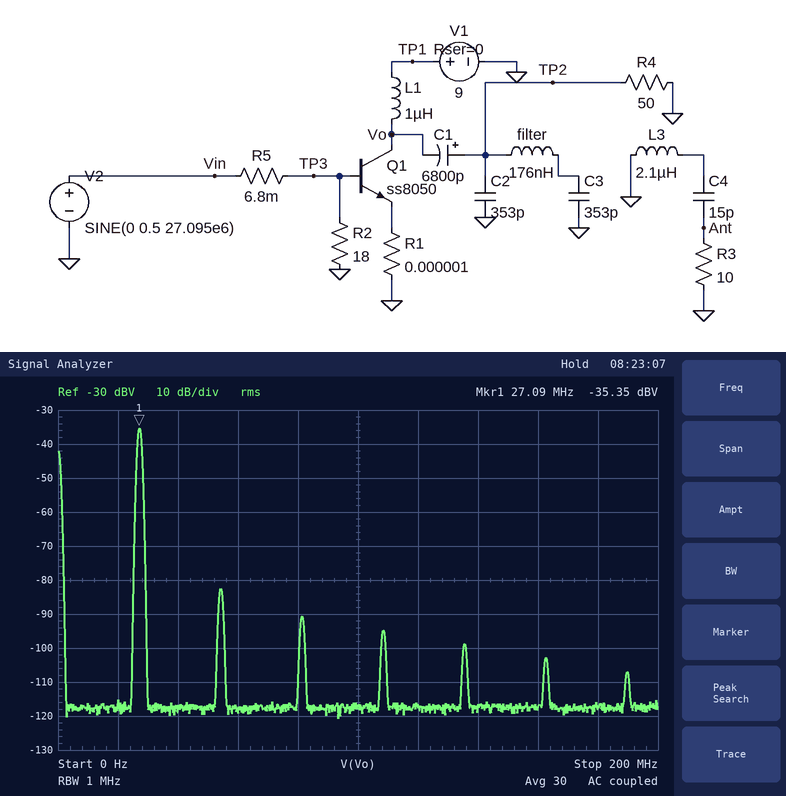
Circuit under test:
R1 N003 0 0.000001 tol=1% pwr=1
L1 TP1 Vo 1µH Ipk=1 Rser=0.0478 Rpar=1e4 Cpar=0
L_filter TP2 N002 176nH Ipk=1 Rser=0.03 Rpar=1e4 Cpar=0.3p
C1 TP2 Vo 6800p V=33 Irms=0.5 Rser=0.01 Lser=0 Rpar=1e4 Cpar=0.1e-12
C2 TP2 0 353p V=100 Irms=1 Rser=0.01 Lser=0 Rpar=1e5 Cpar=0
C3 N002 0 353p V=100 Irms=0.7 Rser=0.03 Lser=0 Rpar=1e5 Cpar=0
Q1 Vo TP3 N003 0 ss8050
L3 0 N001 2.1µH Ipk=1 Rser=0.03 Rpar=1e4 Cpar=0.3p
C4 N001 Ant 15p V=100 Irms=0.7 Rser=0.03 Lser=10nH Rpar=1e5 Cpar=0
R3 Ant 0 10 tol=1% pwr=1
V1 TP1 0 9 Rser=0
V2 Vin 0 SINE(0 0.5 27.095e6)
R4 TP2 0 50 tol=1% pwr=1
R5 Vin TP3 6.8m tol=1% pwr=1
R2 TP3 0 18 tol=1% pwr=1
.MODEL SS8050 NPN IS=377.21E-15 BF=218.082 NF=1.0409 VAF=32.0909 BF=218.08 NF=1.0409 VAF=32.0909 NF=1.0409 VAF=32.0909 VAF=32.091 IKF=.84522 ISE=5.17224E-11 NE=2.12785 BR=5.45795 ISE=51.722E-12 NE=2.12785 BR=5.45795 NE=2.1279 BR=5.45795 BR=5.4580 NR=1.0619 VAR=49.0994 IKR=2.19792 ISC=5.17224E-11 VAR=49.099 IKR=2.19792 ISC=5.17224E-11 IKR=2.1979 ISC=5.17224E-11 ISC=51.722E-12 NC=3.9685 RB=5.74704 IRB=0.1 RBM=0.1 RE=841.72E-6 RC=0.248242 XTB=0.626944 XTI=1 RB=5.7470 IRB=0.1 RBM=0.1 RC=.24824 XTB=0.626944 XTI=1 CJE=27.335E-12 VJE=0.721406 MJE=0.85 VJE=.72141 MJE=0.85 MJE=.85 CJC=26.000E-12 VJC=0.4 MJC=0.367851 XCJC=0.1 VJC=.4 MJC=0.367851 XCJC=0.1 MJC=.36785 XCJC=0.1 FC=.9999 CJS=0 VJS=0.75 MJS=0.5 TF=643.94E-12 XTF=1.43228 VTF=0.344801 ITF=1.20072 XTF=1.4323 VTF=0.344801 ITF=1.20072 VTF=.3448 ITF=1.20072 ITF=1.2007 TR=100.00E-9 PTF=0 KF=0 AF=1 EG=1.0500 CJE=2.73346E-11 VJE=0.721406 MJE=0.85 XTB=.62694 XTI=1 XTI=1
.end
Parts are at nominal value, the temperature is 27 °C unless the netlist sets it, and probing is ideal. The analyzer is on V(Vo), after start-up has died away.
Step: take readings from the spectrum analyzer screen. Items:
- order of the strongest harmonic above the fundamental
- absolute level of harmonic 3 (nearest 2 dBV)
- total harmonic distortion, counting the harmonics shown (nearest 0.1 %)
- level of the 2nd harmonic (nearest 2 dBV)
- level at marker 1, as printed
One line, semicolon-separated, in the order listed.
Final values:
2; -90 dBV; 0.5 %; -82 dBV; -35.35 dBV
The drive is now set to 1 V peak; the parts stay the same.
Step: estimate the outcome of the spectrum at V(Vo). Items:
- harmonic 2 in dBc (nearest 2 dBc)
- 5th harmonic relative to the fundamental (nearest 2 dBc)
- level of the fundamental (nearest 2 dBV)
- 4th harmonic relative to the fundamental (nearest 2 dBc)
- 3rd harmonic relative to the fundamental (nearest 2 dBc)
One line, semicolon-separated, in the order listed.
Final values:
-16 dBc; -34 dBc; 6 dBV; -34 dBc; -34 dBc
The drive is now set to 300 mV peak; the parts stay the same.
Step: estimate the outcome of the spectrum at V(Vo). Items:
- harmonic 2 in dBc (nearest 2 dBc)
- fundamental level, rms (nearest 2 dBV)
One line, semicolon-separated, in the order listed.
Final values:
-54 dBc; -40 dBV
